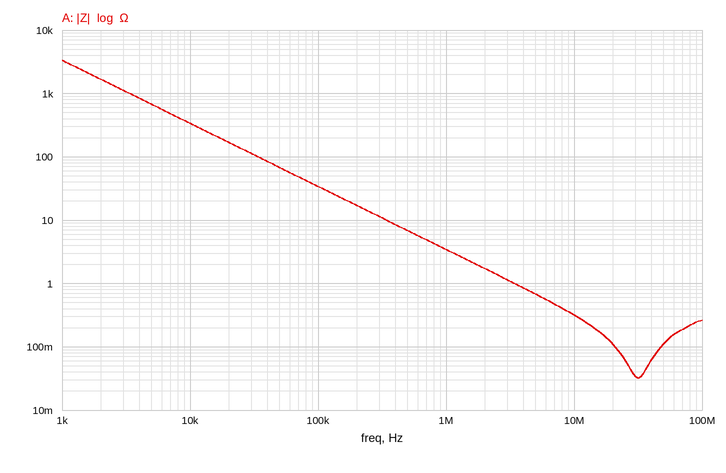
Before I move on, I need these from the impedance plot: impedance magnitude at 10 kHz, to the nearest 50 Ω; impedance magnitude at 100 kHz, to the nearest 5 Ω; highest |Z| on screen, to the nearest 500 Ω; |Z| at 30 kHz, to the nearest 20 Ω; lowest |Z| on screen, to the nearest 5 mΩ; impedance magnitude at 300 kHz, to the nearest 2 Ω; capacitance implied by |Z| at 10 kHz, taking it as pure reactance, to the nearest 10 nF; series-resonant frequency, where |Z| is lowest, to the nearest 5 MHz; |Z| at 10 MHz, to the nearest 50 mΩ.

350 Ω
35 Ω
3.5 kΩ
120 Ω
30 mΩ
12 Ω
50 nF
30 MHz
300 mΩ
